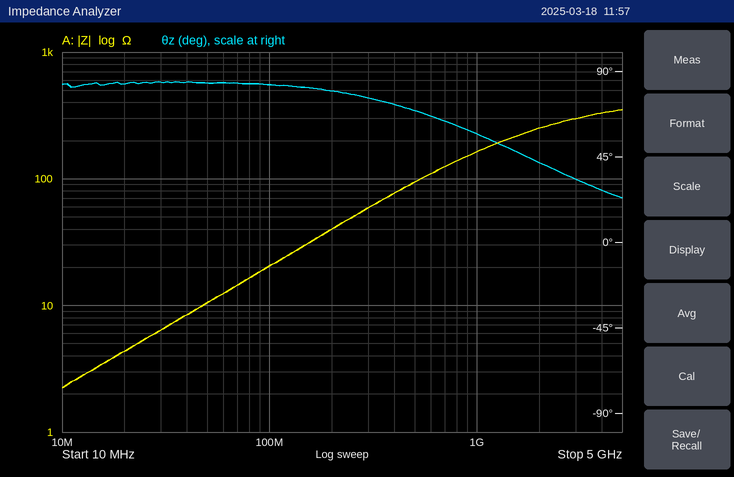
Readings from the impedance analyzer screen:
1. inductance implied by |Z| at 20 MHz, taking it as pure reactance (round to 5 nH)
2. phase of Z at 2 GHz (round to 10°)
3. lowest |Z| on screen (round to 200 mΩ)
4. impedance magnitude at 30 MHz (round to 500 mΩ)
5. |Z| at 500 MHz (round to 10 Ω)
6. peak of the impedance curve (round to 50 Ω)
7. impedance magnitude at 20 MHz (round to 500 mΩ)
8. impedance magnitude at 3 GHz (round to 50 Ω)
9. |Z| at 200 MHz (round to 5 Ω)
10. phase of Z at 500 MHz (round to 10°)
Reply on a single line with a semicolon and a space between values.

35 nH; 40°; 2.2 Ω; 6.5 Ω; 90 Ω; 350 Ω; 4.5 Ω; 300 Ω; 40 Ω; 70°
